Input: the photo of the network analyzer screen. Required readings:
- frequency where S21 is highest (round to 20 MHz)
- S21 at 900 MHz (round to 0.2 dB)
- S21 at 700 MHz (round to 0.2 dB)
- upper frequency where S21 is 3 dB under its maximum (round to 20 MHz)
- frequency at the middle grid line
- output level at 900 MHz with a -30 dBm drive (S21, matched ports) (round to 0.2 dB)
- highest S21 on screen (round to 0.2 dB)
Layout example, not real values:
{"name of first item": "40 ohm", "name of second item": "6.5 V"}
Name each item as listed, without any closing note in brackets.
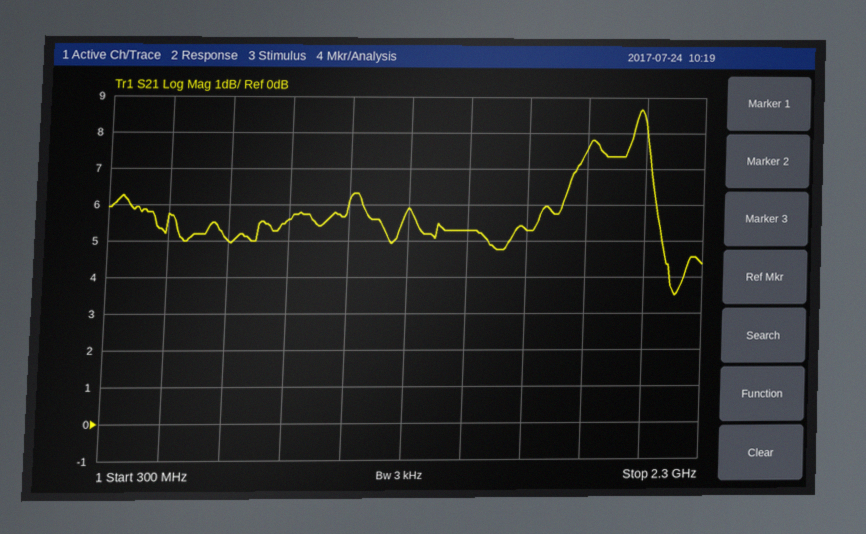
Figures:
{"frequency where S21 is highest": "2.08 GHz", "S21 at 900 MHz": "5.6 dB", "S21 at 700 MHz": "5.0 dB", "upper frequency where S21 is 3 dB under its maximum": "2.14 GHz", "frequency at the middle grid line": "1.3 GHz", "output level at 900 MHz with a -30 dBm drive (S21, matched ports)": "-24.4 dBm", "highest S21 on screen": "8.6 dB"}
